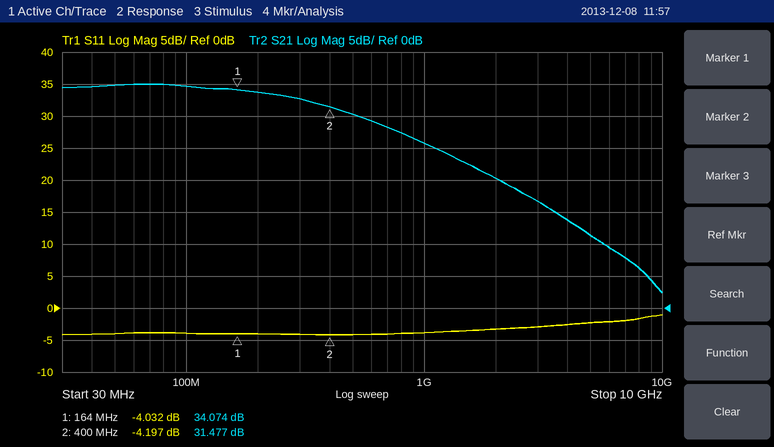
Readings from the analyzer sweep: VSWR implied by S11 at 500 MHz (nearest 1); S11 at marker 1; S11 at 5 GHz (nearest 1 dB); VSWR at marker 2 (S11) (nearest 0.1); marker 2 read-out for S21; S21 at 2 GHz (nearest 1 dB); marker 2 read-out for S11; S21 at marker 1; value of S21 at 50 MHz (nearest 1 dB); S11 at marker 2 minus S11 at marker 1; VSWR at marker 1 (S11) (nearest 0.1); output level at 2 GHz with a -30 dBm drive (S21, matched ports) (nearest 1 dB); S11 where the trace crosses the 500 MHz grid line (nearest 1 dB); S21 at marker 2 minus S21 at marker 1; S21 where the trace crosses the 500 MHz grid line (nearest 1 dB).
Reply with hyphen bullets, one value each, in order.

- 4
- -4.032 dB
- -2 dB
- 4.2
- 31.477 dB
- 20 dB
- -4.197 dB
- 34.074 dB
- 35 dB
- -0.165 dB
- 4.4
- -10 dBm
- -4 dB
- -2.597 dB
- 30 dB
